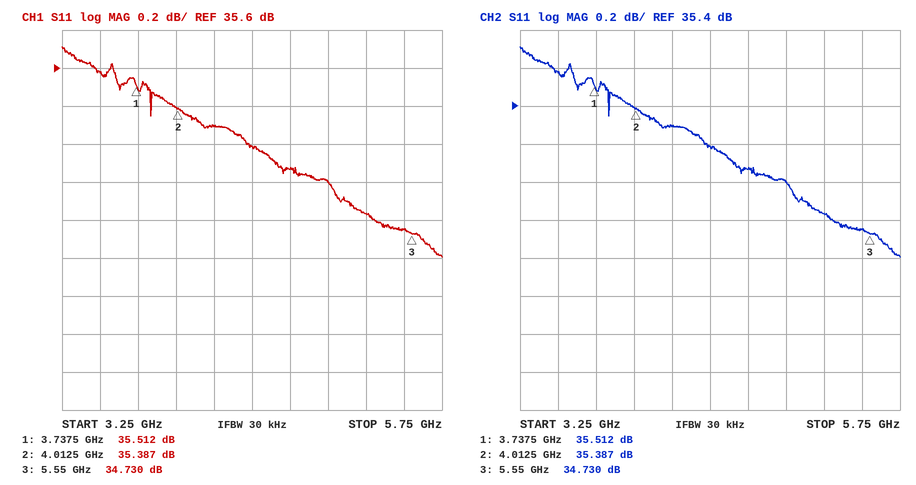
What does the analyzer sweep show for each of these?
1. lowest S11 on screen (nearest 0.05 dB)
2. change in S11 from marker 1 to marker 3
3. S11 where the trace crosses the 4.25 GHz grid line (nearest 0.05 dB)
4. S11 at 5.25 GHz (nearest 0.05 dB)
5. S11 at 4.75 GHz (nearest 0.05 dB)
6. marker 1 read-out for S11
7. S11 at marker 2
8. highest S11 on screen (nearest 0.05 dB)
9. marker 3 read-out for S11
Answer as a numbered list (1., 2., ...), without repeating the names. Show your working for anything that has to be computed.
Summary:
1. 34.60 dB
2. 34.73 − (35.512) = -0.782 dB
3. 35.30 dB
4. 34.85 dB
5. 35.05 dB
6. 35.512 dB
7. 35.387 dB
8. 35.70 dB
9. 34.730 dB
